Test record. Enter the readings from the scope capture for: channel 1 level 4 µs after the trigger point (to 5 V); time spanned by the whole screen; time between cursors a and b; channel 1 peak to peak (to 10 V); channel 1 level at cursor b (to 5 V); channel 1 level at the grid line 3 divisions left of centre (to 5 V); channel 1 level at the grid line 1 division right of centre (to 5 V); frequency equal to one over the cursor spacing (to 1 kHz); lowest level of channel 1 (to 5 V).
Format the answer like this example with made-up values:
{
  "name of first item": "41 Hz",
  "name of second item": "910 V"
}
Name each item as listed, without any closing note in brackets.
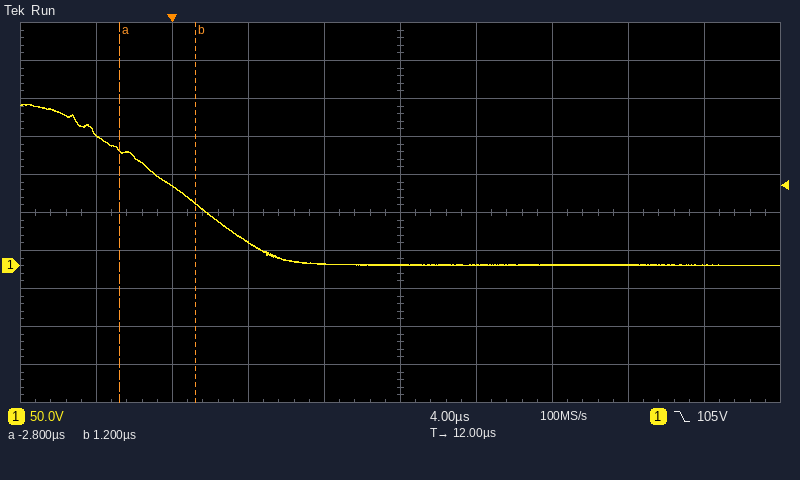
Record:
{
  "channel 1 level 4 µs after the trigger point": "30 V",
  "time spanned by the whole screen": "40 µs",
  "time between cursors a and b": "4.0 µs",
  "channel 1 peak to peak": "210 V",
  "channel 1 level at cursor b": "80 V",
  "channel 1 level at the grid line 3 divisions left of centre": "105 V",
  "channel 1 level at the grid line 1 division right of centre": "0 V",
  "frequency equal to one over the cursor spacing": "250 kHz",
  "lowest level of channel 1": "0 V"
}
